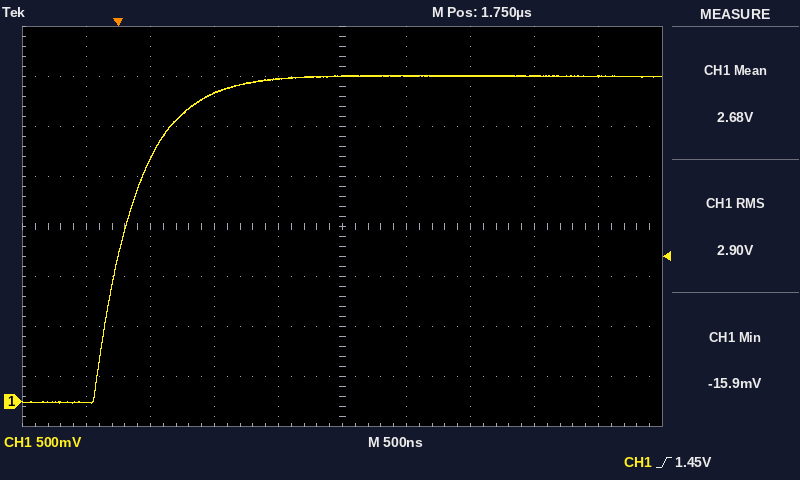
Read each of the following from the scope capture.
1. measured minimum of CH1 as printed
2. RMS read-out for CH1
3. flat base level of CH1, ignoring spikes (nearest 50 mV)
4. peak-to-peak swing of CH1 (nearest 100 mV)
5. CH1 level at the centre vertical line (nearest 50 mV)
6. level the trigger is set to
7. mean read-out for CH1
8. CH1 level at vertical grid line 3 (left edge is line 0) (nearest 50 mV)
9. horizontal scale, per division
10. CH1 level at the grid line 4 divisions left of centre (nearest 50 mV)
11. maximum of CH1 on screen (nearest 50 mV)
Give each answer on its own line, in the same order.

-15.9 mV
2.90 V
0 mV
3.30 V
3.25 V
1.45 V
2.68 V
3.10 V
500 ns
0 mV
3.25 V
